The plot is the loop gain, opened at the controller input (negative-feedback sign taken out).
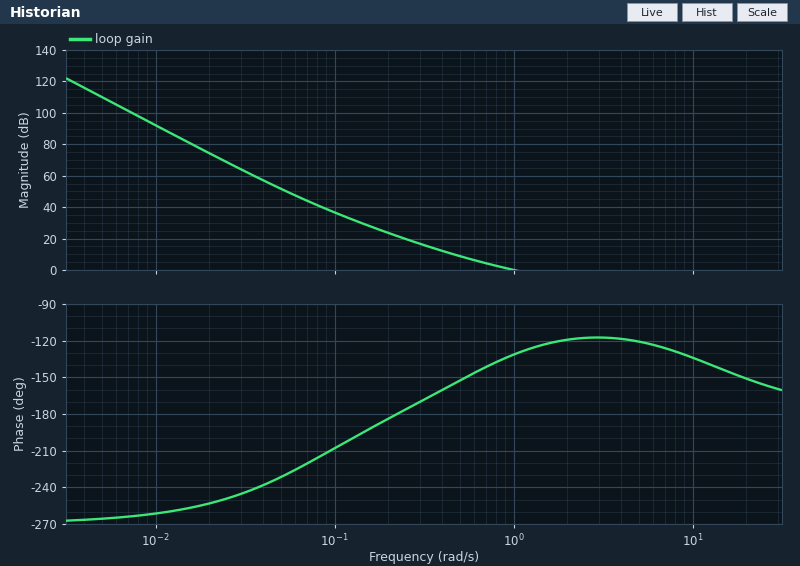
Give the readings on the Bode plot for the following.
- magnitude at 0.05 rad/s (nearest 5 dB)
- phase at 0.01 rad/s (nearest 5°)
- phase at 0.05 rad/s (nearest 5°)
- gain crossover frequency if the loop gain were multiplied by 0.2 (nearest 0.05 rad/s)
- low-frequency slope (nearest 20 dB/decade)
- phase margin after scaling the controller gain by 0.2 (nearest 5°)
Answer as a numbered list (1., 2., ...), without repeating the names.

1. 50 dB
2. -260°
3. -230°
4. 0.35 rad/s
5. -60 dB/decade
6. 15°
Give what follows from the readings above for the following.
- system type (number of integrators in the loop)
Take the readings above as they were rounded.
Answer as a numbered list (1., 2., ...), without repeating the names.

1. 3
